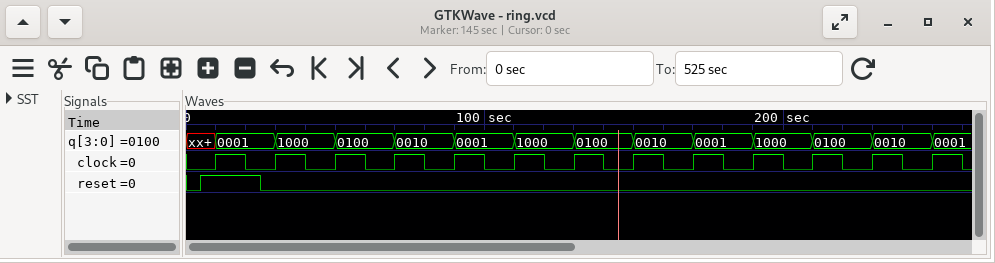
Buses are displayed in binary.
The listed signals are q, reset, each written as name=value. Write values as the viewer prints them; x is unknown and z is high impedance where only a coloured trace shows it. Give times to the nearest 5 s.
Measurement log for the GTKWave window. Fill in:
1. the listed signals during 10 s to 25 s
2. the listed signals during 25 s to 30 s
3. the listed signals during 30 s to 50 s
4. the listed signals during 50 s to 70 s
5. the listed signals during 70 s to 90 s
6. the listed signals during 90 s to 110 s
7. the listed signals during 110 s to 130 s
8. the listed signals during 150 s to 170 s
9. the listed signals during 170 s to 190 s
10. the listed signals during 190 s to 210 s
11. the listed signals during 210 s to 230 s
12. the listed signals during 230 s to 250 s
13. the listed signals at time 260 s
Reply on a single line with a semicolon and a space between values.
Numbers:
q=0001, reset=1; q=0001, reset=0; q=1000, reset=0; q=0100, reset=0; q=0010, reset=0; q=0001, reset=0; q=1000, reset=0; q=0010, reset=0; q=0001, reset=0; q=1000, reset=0; q=0100, reset=0; q=0010, reset=0; q=0001, reset=0
